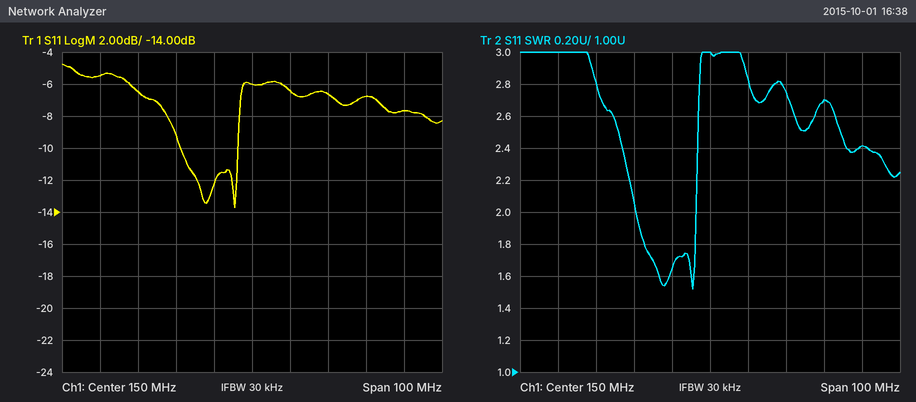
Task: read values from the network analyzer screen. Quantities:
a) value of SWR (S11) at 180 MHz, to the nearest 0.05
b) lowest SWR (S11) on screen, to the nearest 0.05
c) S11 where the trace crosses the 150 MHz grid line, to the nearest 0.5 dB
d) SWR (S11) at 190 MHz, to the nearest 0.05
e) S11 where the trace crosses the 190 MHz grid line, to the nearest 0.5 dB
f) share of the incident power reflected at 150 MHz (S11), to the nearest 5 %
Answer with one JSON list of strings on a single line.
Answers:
["2.70", "1.50", "-6.0 dB", "2.40", "-7.5 dB", "25 %"]
